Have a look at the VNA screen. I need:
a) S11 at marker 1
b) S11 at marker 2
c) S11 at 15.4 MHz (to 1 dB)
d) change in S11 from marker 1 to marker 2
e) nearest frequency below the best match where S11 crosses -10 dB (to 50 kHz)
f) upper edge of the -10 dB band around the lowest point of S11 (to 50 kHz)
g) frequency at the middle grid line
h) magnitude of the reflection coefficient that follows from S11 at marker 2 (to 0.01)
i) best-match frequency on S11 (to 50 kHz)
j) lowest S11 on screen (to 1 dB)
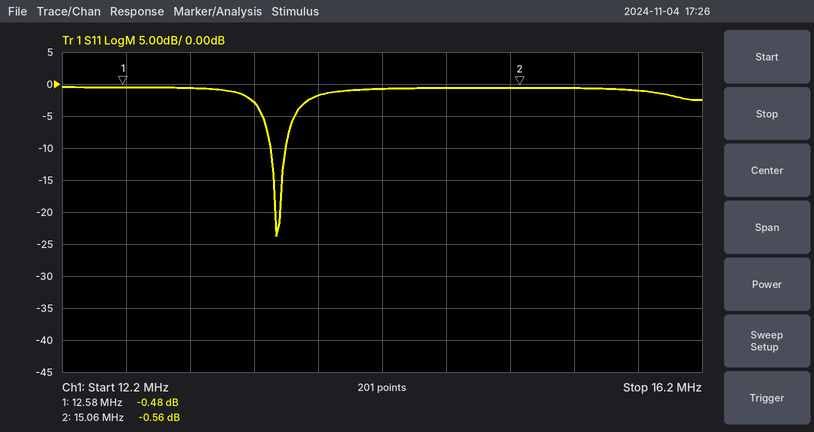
-0.48 dB
-0.56 dB
-1 dB
-0.08 dB
13.50 MHz
13.60 MHz
14.2 MHz
0.94
13.55 MHz
-24 dB
